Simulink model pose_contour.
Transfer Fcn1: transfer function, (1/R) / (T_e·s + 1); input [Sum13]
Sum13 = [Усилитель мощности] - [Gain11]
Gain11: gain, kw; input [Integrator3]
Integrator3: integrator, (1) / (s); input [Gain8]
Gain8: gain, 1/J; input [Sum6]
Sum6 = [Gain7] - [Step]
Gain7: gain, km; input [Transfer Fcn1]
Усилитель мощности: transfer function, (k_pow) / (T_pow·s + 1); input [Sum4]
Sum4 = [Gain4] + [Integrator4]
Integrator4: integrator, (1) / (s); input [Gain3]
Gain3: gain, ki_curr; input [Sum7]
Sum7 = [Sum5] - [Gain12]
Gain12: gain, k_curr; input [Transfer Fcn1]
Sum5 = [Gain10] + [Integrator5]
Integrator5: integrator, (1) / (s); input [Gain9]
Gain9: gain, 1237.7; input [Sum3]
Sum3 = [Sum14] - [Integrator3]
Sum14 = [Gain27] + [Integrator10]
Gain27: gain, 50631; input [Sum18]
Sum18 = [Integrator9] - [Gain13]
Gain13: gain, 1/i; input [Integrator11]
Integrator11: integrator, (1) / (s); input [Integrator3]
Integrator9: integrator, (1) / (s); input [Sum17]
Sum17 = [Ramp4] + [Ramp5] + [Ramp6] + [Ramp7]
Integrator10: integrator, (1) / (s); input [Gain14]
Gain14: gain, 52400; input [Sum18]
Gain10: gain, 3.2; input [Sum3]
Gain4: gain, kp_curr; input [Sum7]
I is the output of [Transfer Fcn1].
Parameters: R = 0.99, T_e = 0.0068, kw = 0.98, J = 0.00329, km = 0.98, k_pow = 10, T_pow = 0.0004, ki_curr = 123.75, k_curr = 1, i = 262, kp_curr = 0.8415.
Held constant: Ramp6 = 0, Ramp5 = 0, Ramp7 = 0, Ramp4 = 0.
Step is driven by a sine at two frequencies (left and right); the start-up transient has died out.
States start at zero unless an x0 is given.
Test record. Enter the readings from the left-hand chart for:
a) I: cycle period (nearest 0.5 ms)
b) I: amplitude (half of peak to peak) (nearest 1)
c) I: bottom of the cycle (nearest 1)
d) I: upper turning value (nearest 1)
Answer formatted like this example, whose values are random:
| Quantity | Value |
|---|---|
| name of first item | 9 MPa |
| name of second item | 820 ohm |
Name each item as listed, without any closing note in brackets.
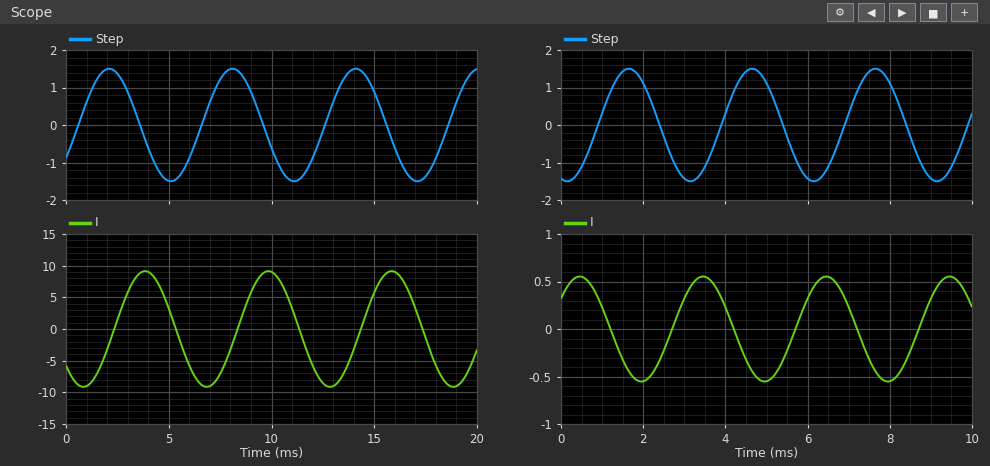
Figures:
| Quantity | Value |
|---|---|
| I: cycle period | 6.0 ms |
| I: amplitude (half of peak to peak) | 9 |
| I: bottom of the cycle | -9 |
| I: upper turning value | 9 |
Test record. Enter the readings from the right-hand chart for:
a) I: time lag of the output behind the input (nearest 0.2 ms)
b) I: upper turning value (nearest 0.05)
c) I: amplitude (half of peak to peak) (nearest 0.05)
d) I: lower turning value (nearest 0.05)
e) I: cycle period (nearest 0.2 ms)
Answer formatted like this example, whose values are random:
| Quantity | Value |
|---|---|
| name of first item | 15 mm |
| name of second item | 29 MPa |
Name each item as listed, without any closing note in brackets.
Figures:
| Quantity | Value |
|---|---|
| I: time lag of the output behind the input | 1.8 ms |
| I: upper turning value | 0.55 |
| I: amplitude (half of peak to peak) | 0.55 |
| I: lower turning value | -0.55 |
| I: cycle period | 3.0 ms |
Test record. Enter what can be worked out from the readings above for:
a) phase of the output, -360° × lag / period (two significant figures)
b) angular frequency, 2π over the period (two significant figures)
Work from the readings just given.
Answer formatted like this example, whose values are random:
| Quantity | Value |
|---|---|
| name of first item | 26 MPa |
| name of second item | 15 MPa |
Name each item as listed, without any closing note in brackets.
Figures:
| Quantity | Value |
|---|---|
| phase of the output, -360° × lag / period | -220° |
| angular frequency, 2π over the period | 2.1 rad/ms |
